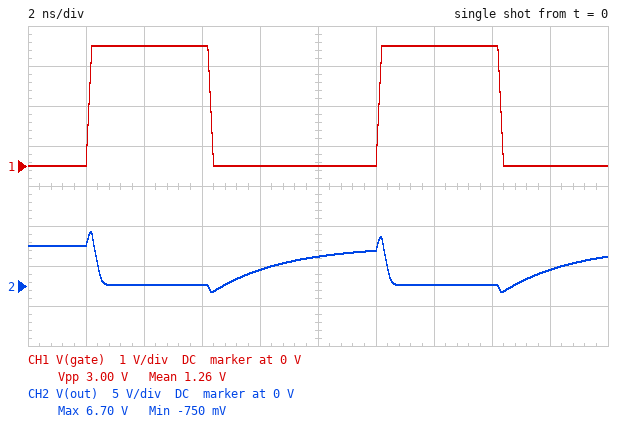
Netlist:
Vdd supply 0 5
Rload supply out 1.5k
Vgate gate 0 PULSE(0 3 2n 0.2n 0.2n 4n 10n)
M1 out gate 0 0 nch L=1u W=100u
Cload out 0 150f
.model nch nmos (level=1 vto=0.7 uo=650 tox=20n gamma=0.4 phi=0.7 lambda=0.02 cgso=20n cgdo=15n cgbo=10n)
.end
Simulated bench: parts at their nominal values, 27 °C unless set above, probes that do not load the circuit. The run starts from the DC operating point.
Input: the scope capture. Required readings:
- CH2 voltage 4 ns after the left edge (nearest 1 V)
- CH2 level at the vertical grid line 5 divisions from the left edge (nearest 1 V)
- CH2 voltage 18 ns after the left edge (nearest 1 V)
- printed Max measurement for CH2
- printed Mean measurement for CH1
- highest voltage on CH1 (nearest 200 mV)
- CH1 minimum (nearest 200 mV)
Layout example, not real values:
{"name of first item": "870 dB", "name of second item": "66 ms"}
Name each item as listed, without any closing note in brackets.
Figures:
{"CH2 voltage 4 ns after the left edge": "0 V", "CH2 level at the vertical grid line 5 divisions from the left edge": "4 V", "CH2 voltage 18 ns after the left edge": "2 V", "printed Max measurement for CH2": "6.70 V", "printed Mean measurement for CH1": "1.26 V", "highest voltage on CH1": "3.0 V", "CH1 minimum": "0 V"}
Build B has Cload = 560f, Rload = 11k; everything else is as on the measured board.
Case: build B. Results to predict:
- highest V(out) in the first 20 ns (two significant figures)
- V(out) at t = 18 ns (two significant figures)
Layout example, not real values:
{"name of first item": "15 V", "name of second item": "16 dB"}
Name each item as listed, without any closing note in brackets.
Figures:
{"highest V(out) in the first 20 ns": "6.4 V", "V(out) at t = 18 ns": "-260 mV"}
